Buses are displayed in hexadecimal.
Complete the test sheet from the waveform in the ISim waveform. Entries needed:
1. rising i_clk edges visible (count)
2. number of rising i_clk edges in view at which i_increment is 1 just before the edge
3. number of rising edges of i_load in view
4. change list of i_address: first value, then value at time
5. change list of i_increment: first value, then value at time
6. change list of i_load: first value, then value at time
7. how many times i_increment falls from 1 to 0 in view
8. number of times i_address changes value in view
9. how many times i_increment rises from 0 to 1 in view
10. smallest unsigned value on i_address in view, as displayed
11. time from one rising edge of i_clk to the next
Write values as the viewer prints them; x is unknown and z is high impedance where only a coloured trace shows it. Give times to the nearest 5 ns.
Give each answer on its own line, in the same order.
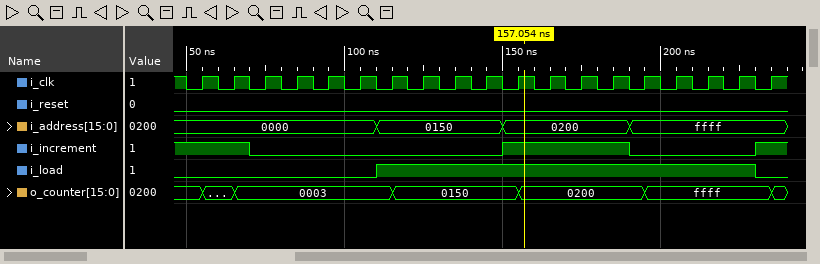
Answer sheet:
19
7
1
0000, 0150 at 110 ns, 0200 at 150 ns, ffff at 190 ns
1, 0 at 70 ns, 1 at 150 ns, 0 at 190 ns, 1 at 230 ns
0, 1 at 110 ns, 0 at 230 ns
2
3
2
0000
10 ns
